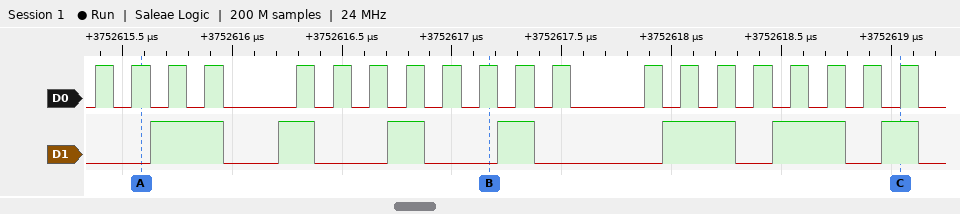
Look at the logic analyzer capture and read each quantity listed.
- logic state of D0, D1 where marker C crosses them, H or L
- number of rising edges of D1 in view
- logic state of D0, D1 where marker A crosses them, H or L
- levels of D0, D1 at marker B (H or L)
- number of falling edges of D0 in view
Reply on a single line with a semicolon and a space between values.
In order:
D0=H, D1=H; 7; D0=H, D1=L; D0=H, D1=L; 20
